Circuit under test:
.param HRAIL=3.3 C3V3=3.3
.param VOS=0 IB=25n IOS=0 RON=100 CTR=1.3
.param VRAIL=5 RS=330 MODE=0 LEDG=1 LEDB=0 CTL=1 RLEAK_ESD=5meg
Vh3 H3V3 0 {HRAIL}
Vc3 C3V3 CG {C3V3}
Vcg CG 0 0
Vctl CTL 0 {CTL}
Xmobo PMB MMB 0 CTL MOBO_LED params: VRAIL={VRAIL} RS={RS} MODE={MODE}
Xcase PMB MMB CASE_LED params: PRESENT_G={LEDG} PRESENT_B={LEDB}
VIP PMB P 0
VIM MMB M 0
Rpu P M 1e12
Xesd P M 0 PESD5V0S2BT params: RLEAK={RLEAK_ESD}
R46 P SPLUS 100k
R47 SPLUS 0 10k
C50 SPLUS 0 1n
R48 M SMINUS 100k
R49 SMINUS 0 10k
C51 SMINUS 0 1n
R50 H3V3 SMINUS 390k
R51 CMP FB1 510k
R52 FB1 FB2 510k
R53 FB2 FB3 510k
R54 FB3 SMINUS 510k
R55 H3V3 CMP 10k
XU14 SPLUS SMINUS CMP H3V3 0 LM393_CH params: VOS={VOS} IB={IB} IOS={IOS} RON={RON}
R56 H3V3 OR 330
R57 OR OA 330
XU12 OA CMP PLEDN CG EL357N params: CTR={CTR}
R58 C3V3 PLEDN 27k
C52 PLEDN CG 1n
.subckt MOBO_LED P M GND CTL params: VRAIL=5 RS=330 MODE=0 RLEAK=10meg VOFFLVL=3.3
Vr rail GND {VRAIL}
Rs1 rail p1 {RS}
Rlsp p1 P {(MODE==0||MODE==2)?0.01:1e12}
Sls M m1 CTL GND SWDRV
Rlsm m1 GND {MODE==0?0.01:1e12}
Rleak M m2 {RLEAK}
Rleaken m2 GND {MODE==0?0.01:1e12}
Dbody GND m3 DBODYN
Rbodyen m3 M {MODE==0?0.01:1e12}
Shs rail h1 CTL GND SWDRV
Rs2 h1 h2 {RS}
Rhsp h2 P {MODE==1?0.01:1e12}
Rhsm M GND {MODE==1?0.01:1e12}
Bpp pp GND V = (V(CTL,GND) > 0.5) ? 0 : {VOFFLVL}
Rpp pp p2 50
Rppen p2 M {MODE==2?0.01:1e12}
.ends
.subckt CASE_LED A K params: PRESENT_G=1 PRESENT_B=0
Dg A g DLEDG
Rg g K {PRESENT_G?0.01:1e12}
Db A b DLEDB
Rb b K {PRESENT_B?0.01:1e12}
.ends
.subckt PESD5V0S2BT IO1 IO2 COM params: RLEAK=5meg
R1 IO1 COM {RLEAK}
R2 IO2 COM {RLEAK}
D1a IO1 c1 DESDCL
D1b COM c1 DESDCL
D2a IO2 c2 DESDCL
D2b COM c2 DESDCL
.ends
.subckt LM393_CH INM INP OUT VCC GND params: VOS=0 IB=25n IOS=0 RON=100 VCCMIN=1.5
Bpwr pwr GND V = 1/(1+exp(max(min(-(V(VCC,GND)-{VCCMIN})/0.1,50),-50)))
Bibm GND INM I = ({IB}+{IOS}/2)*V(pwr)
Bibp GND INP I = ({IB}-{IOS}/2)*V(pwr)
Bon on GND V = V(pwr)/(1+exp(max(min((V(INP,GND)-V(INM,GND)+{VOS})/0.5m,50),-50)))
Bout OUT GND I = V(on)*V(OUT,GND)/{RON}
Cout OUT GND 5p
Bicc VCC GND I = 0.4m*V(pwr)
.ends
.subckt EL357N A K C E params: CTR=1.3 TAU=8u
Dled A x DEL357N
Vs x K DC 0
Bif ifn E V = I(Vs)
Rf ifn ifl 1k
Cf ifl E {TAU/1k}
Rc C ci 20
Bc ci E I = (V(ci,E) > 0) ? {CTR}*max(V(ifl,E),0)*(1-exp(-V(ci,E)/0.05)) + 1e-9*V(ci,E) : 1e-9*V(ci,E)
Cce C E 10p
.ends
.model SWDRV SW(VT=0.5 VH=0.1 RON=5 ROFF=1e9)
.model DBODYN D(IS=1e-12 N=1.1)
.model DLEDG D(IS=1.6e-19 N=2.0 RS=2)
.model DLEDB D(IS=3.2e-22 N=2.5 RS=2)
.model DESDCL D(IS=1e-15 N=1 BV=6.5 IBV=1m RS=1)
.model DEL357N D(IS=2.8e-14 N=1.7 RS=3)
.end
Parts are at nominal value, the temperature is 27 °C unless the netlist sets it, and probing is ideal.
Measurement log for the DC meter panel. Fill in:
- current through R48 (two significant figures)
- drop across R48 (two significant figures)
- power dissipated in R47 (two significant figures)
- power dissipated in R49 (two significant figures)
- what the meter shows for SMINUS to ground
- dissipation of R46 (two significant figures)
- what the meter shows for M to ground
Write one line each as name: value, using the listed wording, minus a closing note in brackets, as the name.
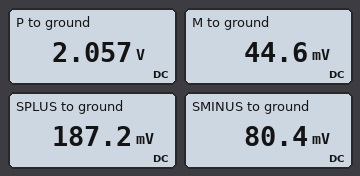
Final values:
current through R48: 360 nA
drop across R48: 36 mV
power dissipated in R47: 3.5 µW
power dissipated in R49: 650 nW
what the meter shows for SMINUS to ground: 80.4 mV
dissipation of R46: 35 µW
what the meter shows for M to ground: 44.6 mV
